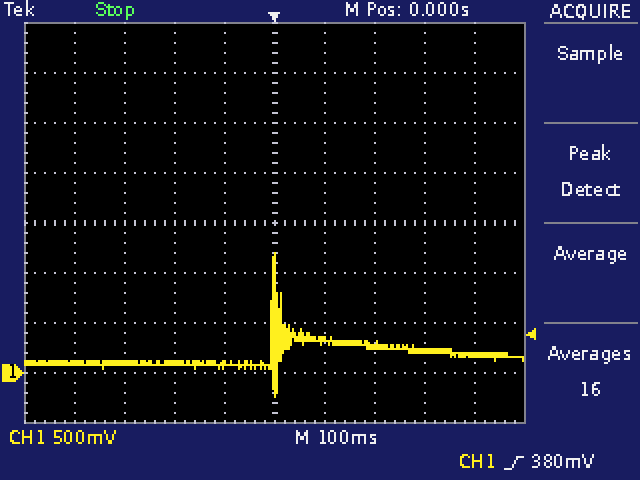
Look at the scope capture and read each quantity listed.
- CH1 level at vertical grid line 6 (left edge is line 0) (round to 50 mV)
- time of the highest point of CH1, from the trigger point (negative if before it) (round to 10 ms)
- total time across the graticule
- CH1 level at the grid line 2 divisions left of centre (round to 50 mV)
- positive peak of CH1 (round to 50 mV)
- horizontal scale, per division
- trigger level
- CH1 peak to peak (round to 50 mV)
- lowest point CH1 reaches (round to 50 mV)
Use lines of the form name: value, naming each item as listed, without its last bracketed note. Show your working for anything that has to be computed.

CH1 level at vertical grid line 6 (left edge is line 0): 300 mV
time of the highest point of CH1, from the trigger point (negative if before it): 0 ms
total time across the graticule: 1 s
CH1 level at the grid line 2 divisions left of centre: 100 mV
positive peak of CH1: 1.20 V
horizontal scale, per division: 100 ms
trigger level: 380 mV
CH1 peak to peak: 1.20 V − (-250 mV) = 1.45 V
lowest point CH1 reaches: -250 mV
